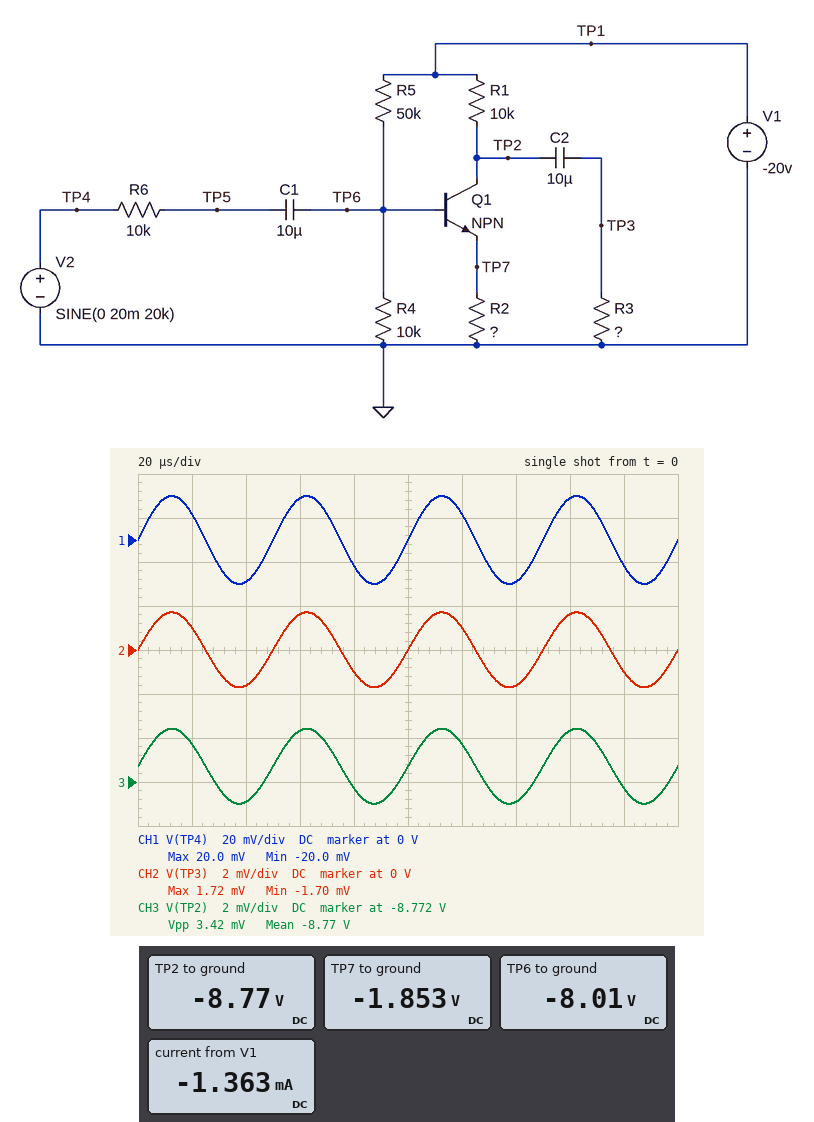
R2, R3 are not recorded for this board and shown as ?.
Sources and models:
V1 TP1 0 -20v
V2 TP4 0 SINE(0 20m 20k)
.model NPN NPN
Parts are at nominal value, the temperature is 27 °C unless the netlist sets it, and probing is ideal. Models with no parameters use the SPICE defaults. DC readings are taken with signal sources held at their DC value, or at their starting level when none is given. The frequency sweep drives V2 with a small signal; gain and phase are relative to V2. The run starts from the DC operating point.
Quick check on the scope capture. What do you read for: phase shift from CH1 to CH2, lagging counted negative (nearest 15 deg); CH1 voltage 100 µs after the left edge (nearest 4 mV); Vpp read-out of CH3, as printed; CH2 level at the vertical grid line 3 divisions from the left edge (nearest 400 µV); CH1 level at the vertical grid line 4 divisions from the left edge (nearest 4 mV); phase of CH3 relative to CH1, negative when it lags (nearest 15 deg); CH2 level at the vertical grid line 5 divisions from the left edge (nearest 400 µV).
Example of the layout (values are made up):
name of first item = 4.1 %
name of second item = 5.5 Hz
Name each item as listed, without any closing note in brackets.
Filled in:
phase shift from CH1 to CH2, lagging counted negative = 0 deg
CH1 voltage 100 µs after the left edge = 0 V
Vpp read-out of CH3, as printed = 3.42 mV
CH2 level at the vertical grid line 3 divisions from the left edge = 1.6 mV
CH1 level at the vertical grid line 4 divisions from the left edge = -12 mV
phase of CH3 relative to CH1, negative when it lags = 0 deg
CH2 level at the vertical grid line 5 divisions from the left edge = 0 V
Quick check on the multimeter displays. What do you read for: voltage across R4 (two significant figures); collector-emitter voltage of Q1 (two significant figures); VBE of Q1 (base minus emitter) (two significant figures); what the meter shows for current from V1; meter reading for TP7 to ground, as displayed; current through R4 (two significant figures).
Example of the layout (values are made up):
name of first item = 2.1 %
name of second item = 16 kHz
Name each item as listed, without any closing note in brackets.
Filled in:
voltage across R4 = 8.0 V
collector-emitter voltage of Q1 = -6.9 V
VBE of Q1 (base minus emitter) = -6.2 V
what the meter shows for current from V1 = -1.363 mA
meter reading for TP7 to ground, as displayed = -1.853 V
current through R4 = 800 µA
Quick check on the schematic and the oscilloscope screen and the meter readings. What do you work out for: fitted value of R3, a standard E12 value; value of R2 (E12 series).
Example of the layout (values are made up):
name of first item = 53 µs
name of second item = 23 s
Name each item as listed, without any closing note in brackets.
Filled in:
fitted value of R3, a standard E12 value = 560 Ω
value of R2 = 3.3 kΩ
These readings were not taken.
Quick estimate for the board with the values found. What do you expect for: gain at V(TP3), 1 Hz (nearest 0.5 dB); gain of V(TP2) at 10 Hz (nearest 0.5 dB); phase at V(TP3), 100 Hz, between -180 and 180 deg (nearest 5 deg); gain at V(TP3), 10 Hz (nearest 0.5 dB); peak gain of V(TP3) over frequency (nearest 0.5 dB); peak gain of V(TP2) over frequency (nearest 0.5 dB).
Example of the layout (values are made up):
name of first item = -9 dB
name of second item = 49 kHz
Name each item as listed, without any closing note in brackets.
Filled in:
gain at V(TP3), 1 Hz = -41.0 dB
gain of V(TP2) at 10 Hz = -13.5 dB
phase at V(TP3), 100 Hz, between -180 and 180 deg = 5 deg
gain at V(TP3), 10 Hz = -23.0 dB
peak gain of V(TP3) over frequency = -21.5 dB
peak gain of V(TP2) over frequency = -10.5 dB
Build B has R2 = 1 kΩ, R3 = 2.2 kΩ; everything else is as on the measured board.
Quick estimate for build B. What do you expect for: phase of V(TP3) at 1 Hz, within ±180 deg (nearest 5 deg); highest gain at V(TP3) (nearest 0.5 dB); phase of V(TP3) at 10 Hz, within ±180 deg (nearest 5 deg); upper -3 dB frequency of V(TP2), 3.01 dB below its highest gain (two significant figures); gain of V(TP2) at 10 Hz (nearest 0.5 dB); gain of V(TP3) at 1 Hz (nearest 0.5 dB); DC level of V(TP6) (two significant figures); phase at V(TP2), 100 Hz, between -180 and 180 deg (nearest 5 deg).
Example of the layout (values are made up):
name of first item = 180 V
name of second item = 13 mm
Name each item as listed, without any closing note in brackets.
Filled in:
phase of V(TP3) at 1 Hz, within ±180 deg = 120 deg
highest gain at V(TP3) = -14.0 dB
phase of V(TP3) at 10 Hz, within ±180 deg = 30 deg
upper -3 dB frequency of V(TP2), 3.01 dB below its highest gain = 23 Hz
gain of V(TP2) at 10 Hz = -13.0 dB
gain of V(TP3) at 1 Hz = -29.5 dB
DC level of V(TP6) = -8.0 V
phase at V(TP2), 100 Hz, between -180 and 180 deg = 0 deg
